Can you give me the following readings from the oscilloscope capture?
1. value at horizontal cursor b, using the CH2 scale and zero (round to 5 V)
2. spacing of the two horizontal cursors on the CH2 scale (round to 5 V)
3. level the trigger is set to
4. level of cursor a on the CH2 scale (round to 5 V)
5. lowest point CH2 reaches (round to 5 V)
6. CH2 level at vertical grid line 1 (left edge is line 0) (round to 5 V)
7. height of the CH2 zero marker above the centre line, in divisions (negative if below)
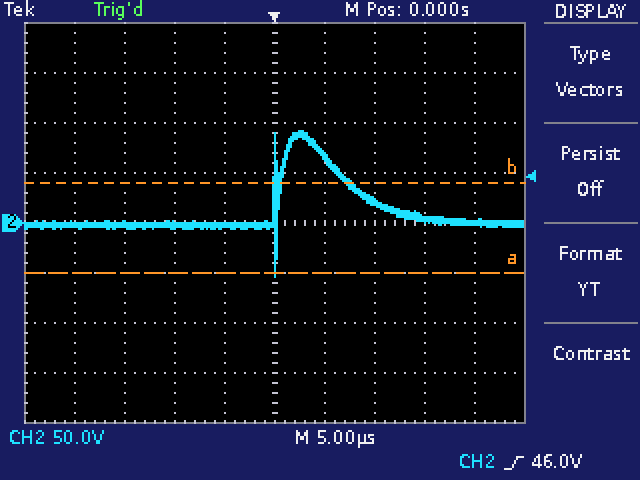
40 V
90 V
46.0 V
-50 V
-55 V
0 V
0.0 div
